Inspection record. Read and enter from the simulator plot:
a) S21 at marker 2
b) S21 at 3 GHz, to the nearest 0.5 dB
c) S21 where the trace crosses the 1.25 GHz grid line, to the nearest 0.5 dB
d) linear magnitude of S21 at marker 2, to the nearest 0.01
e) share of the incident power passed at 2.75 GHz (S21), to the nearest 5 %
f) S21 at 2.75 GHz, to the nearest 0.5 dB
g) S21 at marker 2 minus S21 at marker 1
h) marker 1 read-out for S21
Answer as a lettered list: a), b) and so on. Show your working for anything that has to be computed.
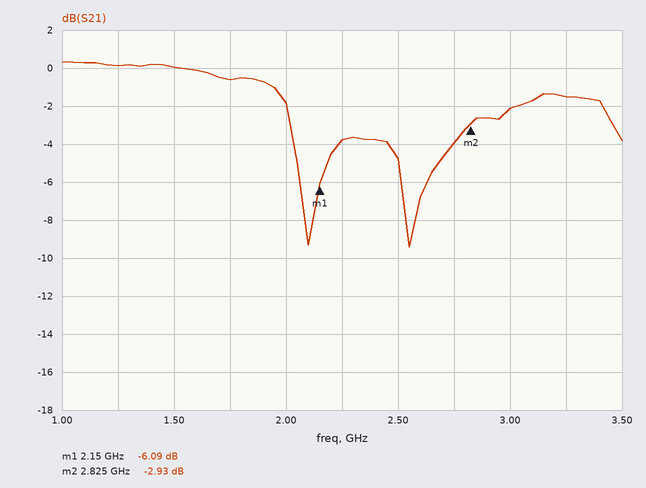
a) -2.93 dB
b) -2.0 dB
c) 0.0 dB
d) 10^(-2.93/20) ≈ 0.71
e) 10^(-4/10) ≈ 40 %
f) -4.0 dB
g) -2.93 − (-6.09) = 3.16 dB
h) -6.09 dB
